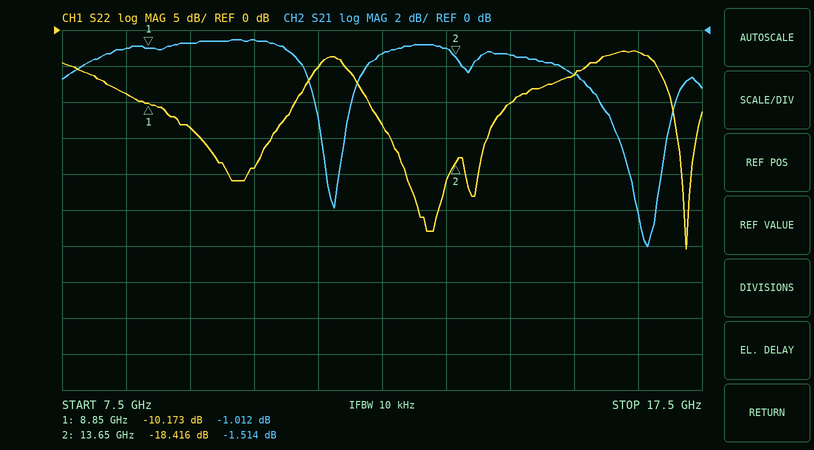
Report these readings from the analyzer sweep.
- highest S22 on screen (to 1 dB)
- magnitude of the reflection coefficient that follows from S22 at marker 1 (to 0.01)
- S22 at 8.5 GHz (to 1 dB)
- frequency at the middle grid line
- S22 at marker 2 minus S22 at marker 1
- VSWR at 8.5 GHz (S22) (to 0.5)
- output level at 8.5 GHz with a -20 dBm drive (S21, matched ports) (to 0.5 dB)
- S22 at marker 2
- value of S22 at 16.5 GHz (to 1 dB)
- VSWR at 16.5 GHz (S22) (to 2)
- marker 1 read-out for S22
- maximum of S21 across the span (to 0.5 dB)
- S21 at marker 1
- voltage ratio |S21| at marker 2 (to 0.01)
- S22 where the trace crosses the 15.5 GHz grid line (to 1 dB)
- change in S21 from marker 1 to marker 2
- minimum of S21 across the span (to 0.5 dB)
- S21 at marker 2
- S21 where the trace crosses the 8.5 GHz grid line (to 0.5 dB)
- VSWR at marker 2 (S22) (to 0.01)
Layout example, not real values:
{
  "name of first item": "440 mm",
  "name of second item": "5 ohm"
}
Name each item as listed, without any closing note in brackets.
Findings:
{
  "highest S22 on screen": "-3 dB",
  "magnitude of the reflection coefficient that follows from S22 at marker 1": "0.31",
  "S22 at 8.5 GHz": "-9 dB",
  "frequency at the middle grid line": "12.5 GHz",
  "S22 at marker 2 minus S22 at marker 1": "-8.243 dB",
  "VSWR at 8.5 GHz (S22)": "2.0",
  "output level at 8.5 GHz with a -20 dBm drive (S21, matched ports)": "-21.0 dBm",
  "S22 at marker 2": "-18.416 dB",
  "value of S22 at 16.5 GHz": "-3 dB",
  "VSWR at 16.5 GHz (S22)": "6",
  "marker 1 read-out for S22": "-10.173 dB",
  "maximum of S21 across the span": "-0.5 dB",
  "S21 at marker 1": "-1.012 dB",
  "voltage ratio |S21| at marker 2": "0.84",
  "S22 where the trace crosses the 15.5 GHz grid line": "-6 dB",
  "change in S21 from marker 1 to marker 2": "-0.502 dB",
  "minimum of S21 across the span": "-12.0 dB",
  "S21 at marker 2": "-1.514 dB",
  "S21 where the trace crosses the 8.5 GHz grid line": "-1.0 dB",
  "VSWR at marker 2 (S22)": "1.27"
}
